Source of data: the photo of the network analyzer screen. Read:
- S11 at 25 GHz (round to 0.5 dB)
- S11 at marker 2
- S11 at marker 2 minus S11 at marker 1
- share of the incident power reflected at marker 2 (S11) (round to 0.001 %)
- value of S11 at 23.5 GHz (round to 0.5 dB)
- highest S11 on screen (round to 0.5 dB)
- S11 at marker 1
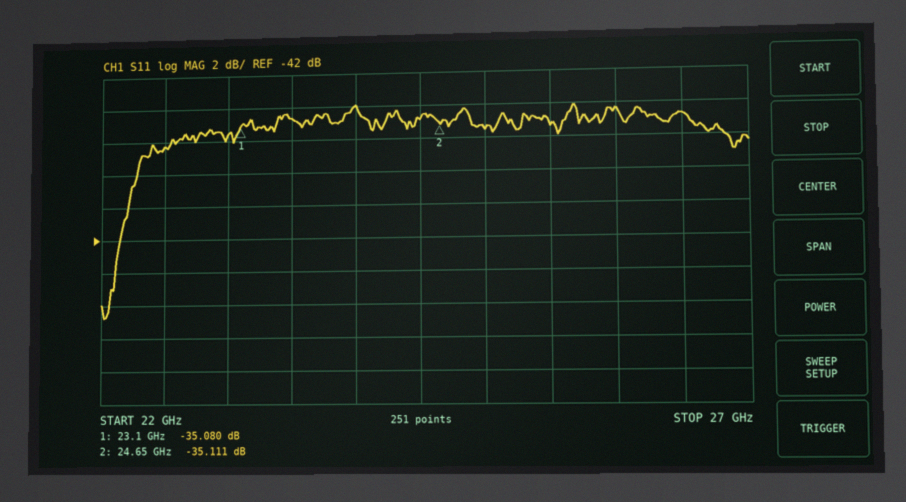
-35.5 dB
-35.111 dB
-0.031 dB
0.031 %
-34.5 dB
-34.0 dB
-35.080 dB
